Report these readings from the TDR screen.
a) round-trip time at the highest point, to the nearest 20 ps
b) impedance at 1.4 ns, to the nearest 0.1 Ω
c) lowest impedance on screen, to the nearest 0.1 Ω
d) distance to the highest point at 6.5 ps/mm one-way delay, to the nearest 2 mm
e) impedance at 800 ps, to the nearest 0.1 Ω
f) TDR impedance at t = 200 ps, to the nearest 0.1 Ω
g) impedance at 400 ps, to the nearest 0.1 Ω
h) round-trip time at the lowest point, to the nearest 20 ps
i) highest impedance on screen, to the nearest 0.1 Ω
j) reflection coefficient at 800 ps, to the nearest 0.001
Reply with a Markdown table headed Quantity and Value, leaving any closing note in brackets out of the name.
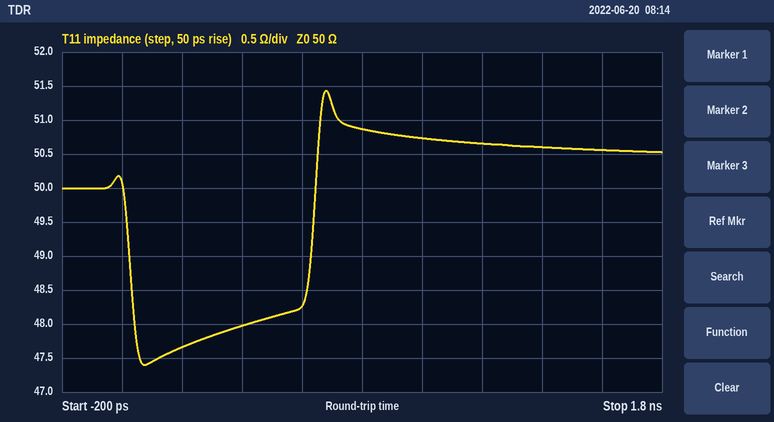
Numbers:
| Quantity | Value |
|---|---|
| round-trip time at the highest point, to the nearest 20 ps | 680 ps |
| impedance at 1.4 ns, to the nearest 0.1 Ω | 50.6 Ω |
| lowest impedance on screen, to the nearest 0.1 Ω | 47.4 Ω |
| distance to the highest point at 6.5 ps/mm one-way delay, to the nearest 2 mm | 52 mm |
| impedance at 800 ps, to the nearest 0.1 Ω | 50.9 Ω |
| TDR impedance at t = 200 ps, to the nearest 0.1 Ω | 47.7 Ω |
| impedance at 400 ps, to the nearest 0.1 Ω | 48.0 Ω |
| round-trip time at the lowest point, to the nearest 20 ps | 80 ps |
| highest impedance on screen, to the nearest 0.1 Ω | 51.4 Ω |
| reflection coefficient at 800 ps, to the nearest 0.001 | +0.009 |
